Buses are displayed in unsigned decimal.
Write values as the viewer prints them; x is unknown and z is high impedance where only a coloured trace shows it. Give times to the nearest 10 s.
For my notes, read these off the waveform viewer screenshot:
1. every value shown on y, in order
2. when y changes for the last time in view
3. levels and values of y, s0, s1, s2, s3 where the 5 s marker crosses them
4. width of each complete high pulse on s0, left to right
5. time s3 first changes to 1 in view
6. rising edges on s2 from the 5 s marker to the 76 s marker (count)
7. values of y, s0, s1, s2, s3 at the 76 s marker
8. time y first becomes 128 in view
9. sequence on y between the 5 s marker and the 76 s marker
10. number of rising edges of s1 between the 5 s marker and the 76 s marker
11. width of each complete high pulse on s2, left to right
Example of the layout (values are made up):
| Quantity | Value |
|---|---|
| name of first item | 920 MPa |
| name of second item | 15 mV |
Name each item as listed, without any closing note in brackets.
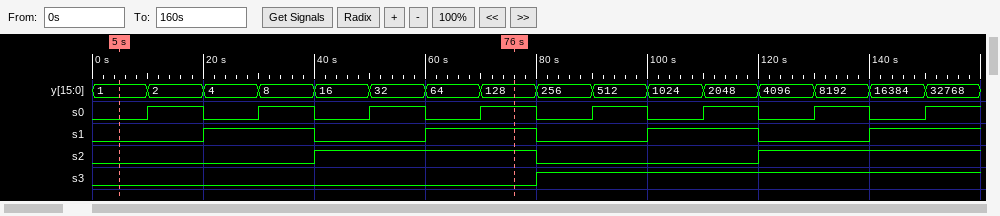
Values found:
| Quantity | Value |
|---|---|
| every value shown on y, in order | 1, 2, 4, 8, 16, 32, 64, 128, 256, 512, 1024, 2048, 4096, 8192, 16384, 32768 |
| when y changes for the last time in view | 150 s |
| levels and values of y, s0, s1, s2, s3 where the 5 s marker crosses them | y=1, s0=0, s1=0, s2=0, s3=0 |
| width of each complete high pulse on s0, left to right | 10 s, 10 s, 10 s, 10 s, 10 s, 10 s, 10 s |
| time s3 first changes to 1 in view | 80 s |
| rising edges on s2 from the 5 s marker to the 76 s marker | 1 |
| values of y, s0, s1, s2, s3 at the 76 s marker | y=128, s0=1, s1=1, s2=1, s3=0 |
| time y first becomes 128 in view | 70 s |
| sequence on y between the 5 s marker and the 76 s marker | 1, 2, 4, 8, 16, 32, 64, 128 |
| number of rising edges of s1 between the 5 s marker and the 76 s marker | 2 |
| width of each complete high pulse on s2, left to right | 40 s |
